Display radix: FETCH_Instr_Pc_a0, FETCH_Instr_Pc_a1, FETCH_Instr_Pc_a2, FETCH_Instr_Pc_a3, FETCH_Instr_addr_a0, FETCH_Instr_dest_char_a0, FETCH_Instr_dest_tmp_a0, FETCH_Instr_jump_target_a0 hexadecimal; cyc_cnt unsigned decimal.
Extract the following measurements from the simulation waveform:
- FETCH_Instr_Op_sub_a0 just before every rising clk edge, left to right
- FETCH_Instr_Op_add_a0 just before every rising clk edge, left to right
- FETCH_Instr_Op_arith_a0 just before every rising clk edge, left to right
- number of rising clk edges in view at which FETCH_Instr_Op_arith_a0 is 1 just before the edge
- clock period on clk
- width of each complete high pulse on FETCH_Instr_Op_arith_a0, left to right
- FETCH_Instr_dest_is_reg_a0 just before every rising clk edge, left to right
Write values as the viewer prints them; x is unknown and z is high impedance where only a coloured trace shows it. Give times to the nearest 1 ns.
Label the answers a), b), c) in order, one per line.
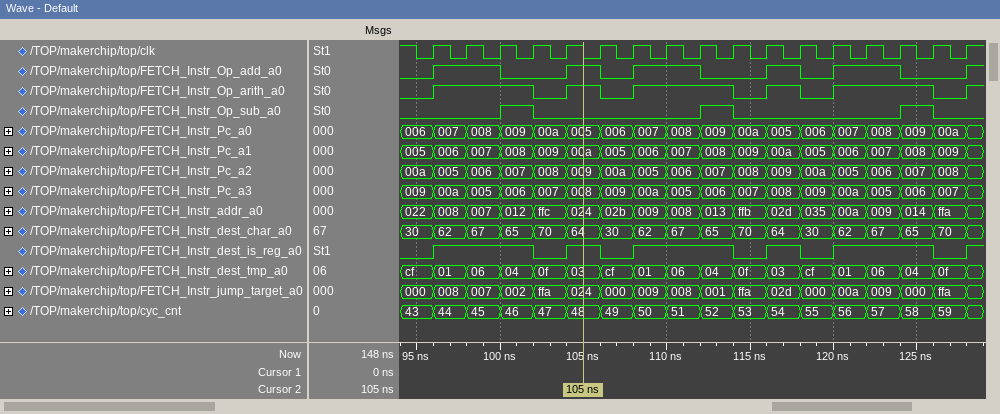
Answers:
a) 0 0 0 1 0 0 0 0 0 1 0 0 0 0 0 1 0
b) 0 1 1 0 0 1 0 1 1 0 0 1 0 1 1 0 0
c) 0 1 1 1 0 1 0 1 1 1 0 1 0 1 1 1 0
d) 11
e) 2 ns
f) 6 ns, 2 ns, 6 ns, 2 ns, 6 ns
g) 0 1 1 1 0 1 0 1 1 1 0 1 0 1 1 1 0
